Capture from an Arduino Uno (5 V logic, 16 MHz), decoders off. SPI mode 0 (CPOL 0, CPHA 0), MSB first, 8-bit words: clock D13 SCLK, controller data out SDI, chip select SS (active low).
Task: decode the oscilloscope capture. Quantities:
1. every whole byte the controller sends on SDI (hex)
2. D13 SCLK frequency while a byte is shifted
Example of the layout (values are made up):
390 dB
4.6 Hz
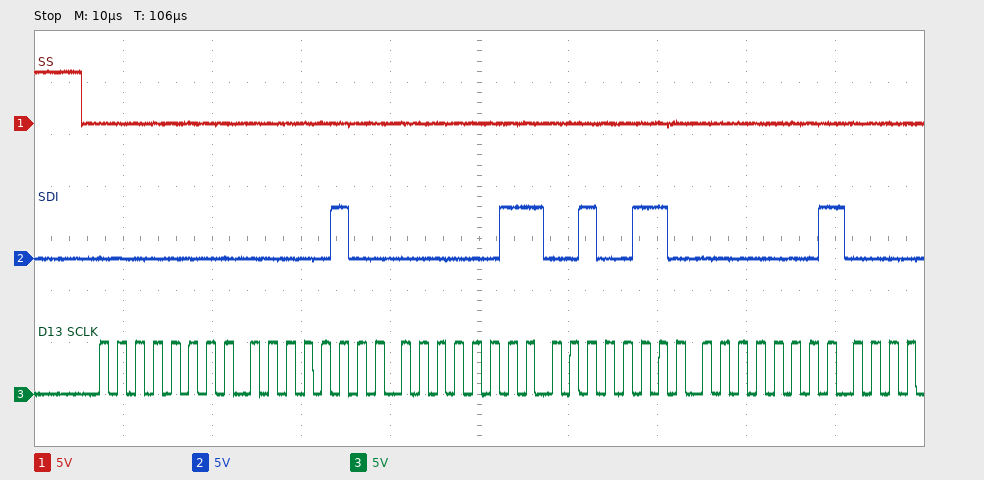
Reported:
00 04 03 26 01
500 kHz
